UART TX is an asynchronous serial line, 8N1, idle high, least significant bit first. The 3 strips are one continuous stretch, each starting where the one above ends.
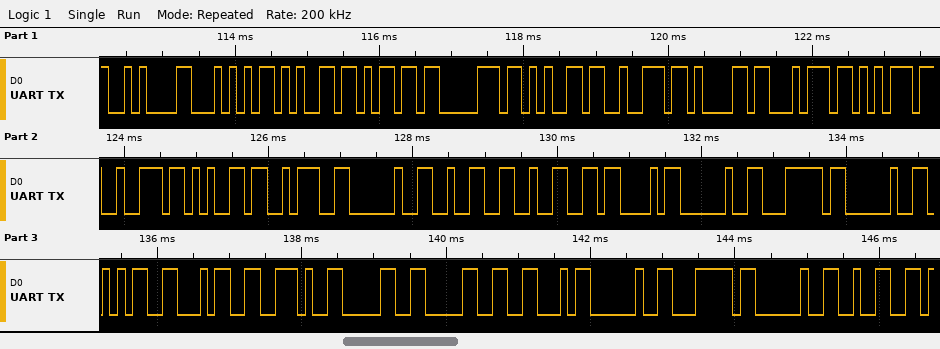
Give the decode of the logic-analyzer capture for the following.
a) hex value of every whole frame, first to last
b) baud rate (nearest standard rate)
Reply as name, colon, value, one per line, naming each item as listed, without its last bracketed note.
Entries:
hex value of every whole frame, first to last: 0A 54 65 6D 70 65 72 61 74 75 72 65 3A 20 32 32 43 20 7C 20 35 34 2E 30 30 46 20 7C 20 32
baud rate: 9600 baud
